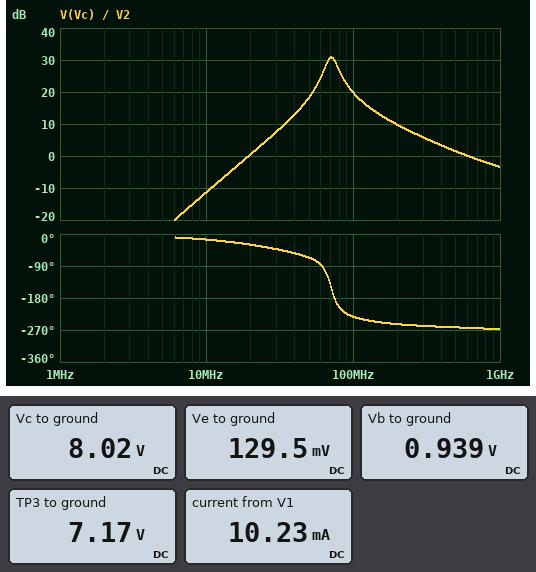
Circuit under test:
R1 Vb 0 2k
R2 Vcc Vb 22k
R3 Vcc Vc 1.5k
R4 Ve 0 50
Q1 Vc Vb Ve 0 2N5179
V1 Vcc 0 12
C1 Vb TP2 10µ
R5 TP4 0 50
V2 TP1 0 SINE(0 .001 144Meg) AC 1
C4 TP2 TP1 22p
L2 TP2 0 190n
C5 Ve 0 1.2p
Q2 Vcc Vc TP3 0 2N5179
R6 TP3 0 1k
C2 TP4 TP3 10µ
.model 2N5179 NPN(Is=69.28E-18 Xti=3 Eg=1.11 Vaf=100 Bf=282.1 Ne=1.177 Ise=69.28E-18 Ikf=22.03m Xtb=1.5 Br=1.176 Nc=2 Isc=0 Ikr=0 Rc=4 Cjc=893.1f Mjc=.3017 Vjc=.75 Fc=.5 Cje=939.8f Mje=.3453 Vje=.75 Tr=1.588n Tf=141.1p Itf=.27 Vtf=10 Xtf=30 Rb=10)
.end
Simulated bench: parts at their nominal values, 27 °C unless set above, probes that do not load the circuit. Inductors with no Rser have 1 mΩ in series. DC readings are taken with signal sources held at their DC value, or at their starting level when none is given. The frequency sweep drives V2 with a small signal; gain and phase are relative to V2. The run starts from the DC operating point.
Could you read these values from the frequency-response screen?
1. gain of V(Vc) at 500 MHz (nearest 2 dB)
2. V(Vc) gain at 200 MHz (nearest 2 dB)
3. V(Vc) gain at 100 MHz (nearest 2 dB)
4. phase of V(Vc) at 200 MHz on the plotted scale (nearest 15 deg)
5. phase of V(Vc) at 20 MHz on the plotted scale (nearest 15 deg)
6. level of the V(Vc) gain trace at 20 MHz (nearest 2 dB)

2 dB
10 dB
20 dB
-255 deg
-30 deg
0 dB
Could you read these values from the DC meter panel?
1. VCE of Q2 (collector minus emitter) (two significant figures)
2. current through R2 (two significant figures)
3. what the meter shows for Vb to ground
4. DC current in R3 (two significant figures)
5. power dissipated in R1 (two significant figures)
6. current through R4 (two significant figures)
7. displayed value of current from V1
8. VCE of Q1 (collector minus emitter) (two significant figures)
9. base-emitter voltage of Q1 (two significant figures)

4.8 V
500 µA
0.939 V
2.7 mA
440 µW
2.6 mA
10.23 mA
7.9 V
810 mV
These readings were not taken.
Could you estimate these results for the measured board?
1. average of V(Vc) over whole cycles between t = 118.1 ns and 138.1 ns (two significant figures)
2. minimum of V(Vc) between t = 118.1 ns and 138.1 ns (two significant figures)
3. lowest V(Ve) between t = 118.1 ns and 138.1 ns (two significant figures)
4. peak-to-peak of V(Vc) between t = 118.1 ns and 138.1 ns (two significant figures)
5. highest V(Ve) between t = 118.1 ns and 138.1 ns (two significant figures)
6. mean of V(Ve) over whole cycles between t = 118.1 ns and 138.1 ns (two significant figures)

8.0 V
8.0 V
130 mV
9.6 mV
130 mV
130 mV
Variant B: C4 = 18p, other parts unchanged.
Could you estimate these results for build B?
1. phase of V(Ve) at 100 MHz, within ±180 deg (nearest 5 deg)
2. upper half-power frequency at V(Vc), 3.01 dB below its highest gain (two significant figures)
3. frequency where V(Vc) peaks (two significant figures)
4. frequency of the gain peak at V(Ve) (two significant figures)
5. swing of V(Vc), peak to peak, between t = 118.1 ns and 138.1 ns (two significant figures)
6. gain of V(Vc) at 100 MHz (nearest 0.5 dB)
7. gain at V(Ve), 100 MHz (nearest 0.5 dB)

25 deg
86 MHz
77 MHz
78 MHz
9.9 mV
21.0 dB
4.0 dB
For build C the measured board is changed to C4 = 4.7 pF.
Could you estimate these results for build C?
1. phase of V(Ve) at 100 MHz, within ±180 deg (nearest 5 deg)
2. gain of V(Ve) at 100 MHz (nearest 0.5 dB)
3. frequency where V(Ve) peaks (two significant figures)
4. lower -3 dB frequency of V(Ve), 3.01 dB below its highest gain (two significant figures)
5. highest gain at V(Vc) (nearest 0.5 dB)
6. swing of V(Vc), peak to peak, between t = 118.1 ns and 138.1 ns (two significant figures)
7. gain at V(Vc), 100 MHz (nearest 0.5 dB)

140 deg
-4.0 dB
130 MHz
110 MHz
17.0 dB
12 mV
13.0 dB
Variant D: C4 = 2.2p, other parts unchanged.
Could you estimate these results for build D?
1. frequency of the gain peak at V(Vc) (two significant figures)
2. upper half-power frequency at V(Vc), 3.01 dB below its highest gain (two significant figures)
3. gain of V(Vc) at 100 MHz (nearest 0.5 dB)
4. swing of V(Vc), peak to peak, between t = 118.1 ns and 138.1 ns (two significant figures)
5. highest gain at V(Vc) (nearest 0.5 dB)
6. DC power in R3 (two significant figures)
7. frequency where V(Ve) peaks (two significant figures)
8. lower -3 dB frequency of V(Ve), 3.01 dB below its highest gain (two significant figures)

150 MHz
200 MHz
4.0 dB
6.1 mV
10.0 dB
11 mW
160 MHz
130 MHz
